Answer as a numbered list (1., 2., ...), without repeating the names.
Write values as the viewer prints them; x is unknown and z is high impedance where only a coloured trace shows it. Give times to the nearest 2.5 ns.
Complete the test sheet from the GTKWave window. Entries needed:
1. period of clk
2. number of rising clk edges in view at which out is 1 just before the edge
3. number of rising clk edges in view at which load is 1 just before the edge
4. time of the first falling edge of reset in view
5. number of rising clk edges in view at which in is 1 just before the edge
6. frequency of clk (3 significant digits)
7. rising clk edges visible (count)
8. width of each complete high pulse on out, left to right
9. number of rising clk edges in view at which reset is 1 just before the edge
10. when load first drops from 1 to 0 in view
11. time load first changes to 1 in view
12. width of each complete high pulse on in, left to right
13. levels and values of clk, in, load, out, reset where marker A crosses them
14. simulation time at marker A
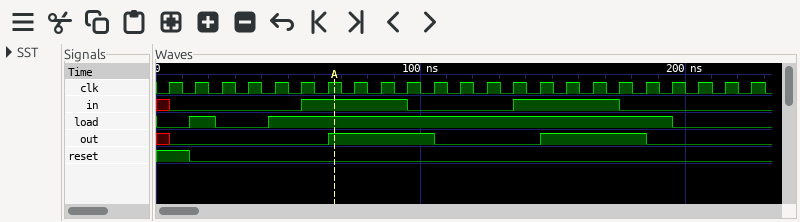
1. 10 ns
2. 8
3. 17
4. 12.5 ns
5. 8
6. 100 MHz
7. 23
8. 40 ns, 40 ns
9. 1
10. 22.5 ns
11. 12.5 ns
12. 40 ns, 40 ns
13. clk=1, in=1, load=1, out=1, reset=0
14. 67.5 ns
